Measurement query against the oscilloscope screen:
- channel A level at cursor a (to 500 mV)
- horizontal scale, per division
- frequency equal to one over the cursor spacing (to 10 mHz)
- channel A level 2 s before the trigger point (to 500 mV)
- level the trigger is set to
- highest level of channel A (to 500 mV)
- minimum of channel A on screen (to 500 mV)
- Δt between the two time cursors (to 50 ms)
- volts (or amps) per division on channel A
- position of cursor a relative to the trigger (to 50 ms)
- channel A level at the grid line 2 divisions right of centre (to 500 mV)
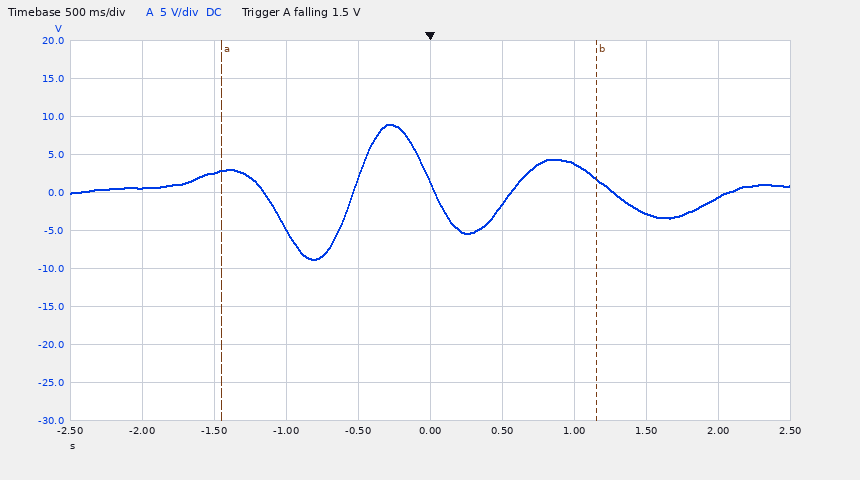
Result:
3.0 V
500 ms
380 mHz
500 mV
1.5 V
9.0 V
-9.0 V
2.60 s
5 V
-1.45 s
4.0 V
